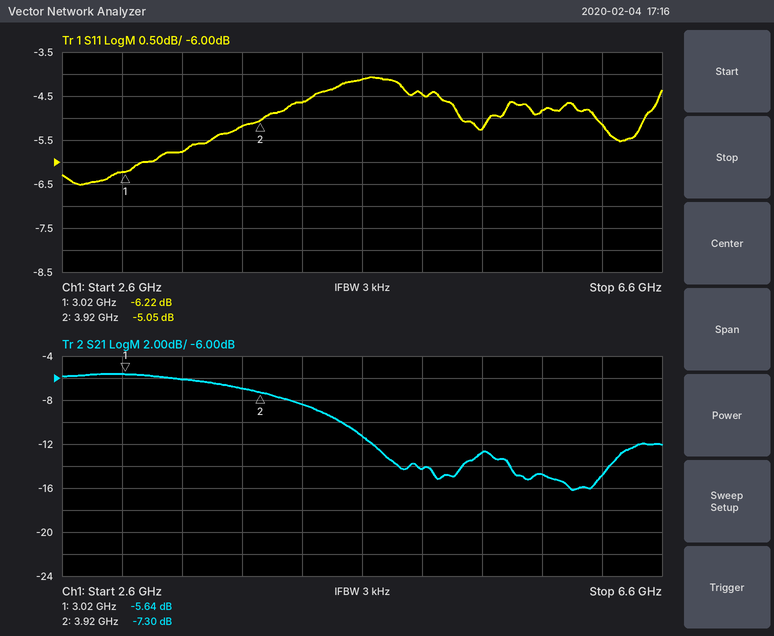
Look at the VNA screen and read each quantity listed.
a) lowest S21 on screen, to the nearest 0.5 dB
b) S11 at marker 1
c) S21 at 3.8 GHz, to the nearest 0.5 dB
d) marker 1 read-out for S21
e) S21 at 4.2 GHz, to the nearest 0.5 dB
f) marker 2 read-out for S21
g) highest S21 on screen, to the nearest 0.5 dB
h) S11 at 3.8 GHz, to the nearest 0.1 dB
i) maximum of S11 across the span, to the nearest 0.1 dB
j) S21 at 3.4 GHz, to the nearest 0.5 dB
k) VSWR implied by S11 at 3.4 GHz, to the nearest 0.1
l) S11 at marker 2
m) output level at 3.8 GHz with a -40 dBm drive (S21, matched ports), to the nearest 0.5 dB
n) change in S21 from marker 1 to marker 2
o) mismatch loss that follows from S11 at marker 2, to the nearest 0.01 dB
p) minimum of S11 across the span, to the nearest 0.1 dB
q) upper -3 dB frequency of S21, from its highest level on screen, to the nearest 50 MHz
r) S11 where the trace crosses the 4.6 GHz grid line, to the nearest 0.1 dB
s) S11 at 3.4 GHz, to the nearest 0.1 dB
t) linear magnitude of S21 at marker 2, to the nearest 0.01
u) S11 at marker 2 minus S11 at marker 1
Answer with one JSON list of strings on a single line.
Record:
["-16.0 dB", "-6.22 dB", "-7.0 dB", "-5.64 dB", "-8.5 dB", "-7.30 dB", "-5.5 dB", "-5.2 dB", "-4.1 dB", "-6.0 dB", "3.1", "-5.05 dB", "-47.0 dBm", "-1.66 dB", "1.63 dB", "-6.5 dB", "4.25 GHz", "-4.1 dB", "-5.8 dB", "0.43", "1.17 dB"]
